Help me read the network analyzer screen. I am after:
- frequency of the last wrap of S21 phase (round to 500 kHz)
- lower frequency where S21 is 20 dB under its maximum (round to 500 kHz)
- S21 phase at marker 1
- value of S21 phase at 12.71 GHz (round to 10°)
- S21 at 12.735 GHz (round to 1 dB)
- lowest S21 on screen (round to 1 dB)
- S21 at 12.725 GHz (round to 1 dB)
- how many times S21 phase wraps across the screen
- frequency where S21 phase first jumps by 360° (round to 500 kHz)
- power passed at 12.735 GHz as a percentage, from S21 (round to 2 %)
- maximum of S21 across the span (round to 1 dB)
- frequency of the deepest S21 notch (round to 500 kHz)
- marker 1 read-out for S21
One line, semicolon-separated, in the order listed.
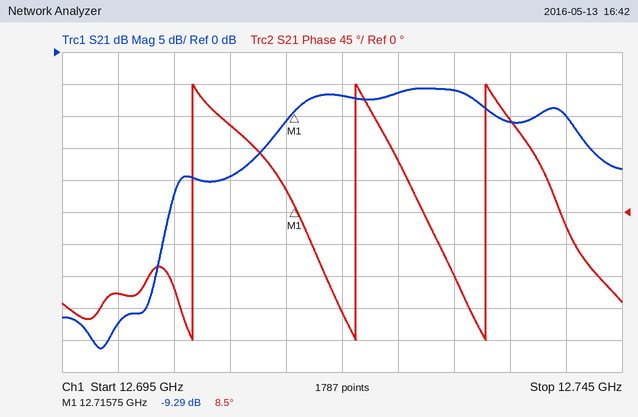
12.7330 GHz; 12.7045 GHz; 8.5°; 120°; -11 dB; -46 dB; -6 dB; 3; 12.7065 GHz; 8 %; -6 dB; 12.6985 GHz; -9.29 dB
